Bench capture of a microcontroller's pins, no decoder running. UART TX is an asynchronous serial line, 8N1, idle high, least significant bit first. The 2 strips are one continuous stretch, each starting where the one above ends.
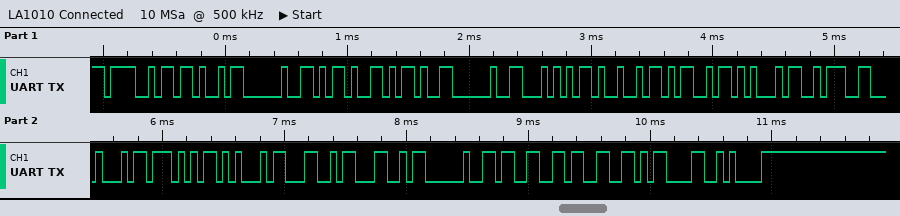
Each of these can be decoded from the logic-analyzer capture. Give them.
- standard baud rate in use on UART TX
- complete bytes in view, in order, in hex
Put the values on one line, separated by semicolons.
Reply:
19200 baud; 4F 4B 20 2D 2D 20 54 49 4D 45 3A 44 57 45 4C 4C 20 33 33 0D 0A
